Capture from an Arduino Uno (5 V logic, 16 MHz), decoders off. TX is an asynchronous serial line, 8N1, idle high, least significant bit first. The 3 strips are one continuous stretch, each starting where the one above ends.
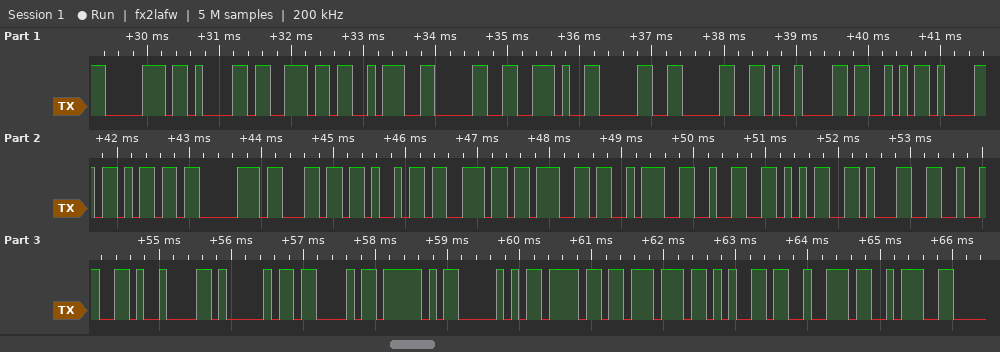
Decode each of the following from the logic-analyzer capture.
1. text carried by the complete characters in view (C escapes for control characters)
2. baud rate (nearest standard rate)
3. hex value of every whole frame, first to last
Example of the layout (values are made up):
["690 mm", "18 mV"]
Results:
["\"pan:0.00\\tSampling:2512\\tAC_Power:\"", "9600 baud", "70 61 6E 3A 30 2E 30 30 09 53 61 6D 70 6C 69 6E 67 3A 32 35 31 32 09 41 43 5F 50 6F 77 65 72 3A"]
